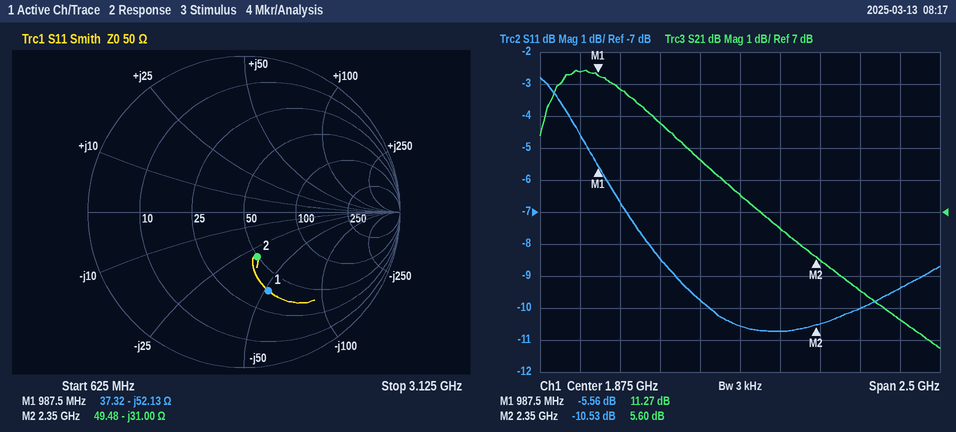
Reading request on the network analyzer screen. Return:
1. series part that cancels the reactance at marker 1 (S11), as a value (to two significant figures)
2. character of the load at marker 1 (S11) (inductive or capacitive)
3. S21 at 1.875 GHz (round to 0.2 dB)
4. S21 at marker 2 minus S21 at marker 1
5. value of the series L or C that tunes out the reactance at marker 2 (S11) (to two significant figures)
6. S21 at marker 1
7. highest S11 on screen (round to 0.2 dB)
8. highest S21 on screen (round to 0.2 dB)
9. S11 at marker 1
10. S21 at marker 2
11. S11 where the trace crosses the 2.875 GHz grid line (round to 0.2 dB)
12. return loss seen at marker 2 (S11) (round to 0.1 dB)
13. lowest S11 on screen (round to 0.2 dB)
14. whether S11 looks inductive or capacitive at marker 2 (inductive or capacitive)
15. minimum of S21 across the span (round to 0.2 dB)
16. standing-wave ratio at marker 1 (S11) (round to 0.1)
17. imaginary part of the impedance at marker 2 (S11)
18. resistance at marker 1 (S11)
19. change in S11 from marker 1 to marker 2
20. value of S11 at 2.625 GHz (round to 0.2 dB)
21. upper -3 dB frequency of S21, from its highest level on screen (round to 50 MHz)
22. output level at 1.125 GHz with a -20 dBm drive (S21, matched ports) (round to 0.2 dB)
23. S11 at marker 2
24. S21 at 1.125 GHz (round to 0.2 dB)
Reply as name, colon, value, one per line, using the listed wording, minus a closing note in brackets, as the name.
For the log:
series part that cancels the reactance at marker 1 (S11), as a value: 8.4 nH
character of the load at marker 1 (S11): capacitive
S21 at 1.875 GHz: 7.6 dB
S21 at marker 2 minus S21 at marker 1: -5.67 dB
value of the series L or C that tunes out the reactance at marker 2 (S11): 2.1 nH
S21 at marker 1: 11.27 dB
highest S11 on screen: -2.8 dB
highest S21 on screen: 11.4 dB
S11 at marker 1: -5.56 dB
S21 at marker 2: 5.60 dB
S11 where the trace crosses the 2.875 GHz grid line: -9.4 dB
return loss seen at marker 2 (S11): 10.5 dB
lowest S11 on screen: -10.8 dB
whether S11 looks inductive or capacitive at marker 2: capacitive
minimum of S21 across the span: 2.8 dB
standing-wave ratio at marker 1 (S11): 3.2
imaginary part of the impedance at marker 2: -31.00 Ω
resistance at marker 1: 37.32 Ω
change in S11 from marker 1 to marker 2: -4.97 dB
value of S11 at 2.625 GHz: -10.0 dB
upper -3 dB frequency of S21, from its highest level on screen: 1.65 GHz
output level at 1.125 GHz with a -20 dBm drive (S21, matched ports): -9.2 dBm
S11 at marker 2: -10.53 dB
S21 at 1.125 GHz: 10.8 dB
